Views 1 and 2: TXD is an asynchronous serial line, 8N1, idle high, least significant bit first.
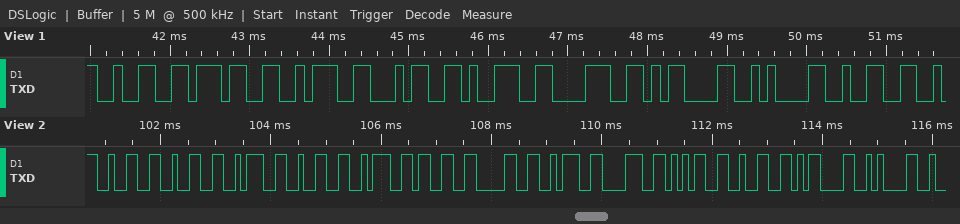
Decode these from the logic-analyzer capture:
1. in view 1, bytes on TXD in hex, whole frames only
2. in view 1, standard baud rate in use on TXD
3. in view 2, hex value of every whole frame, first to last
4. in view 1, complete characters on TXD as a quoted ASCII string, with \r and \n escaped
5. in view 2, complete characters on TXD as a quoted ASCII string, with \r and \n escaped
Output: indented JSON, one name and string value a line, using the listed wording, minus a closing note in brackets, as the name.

{
  "in view 1, bytes on TXD in hex, whole frames only": "32 37 3A 34 39 38 0D 0A 32",
  "in view 1, standard baud rate in use on TXD": "9600 baud",
  "in view 2, hex value of every whole frame, first to last": "32 32 3A 32 3A 33 30 3A 38 35 32 0D 0A",
  "in view 1, complete characters on TXD as a quoted ASCII string, with \\r and \\n escaped": "\"27:498\\r\\n2\"",
  "in view 2, complete characters on TXD as a quoted ASCII string, with \\r and \\n escaped": "\"22:2:30:852\\r\\n\""
}
